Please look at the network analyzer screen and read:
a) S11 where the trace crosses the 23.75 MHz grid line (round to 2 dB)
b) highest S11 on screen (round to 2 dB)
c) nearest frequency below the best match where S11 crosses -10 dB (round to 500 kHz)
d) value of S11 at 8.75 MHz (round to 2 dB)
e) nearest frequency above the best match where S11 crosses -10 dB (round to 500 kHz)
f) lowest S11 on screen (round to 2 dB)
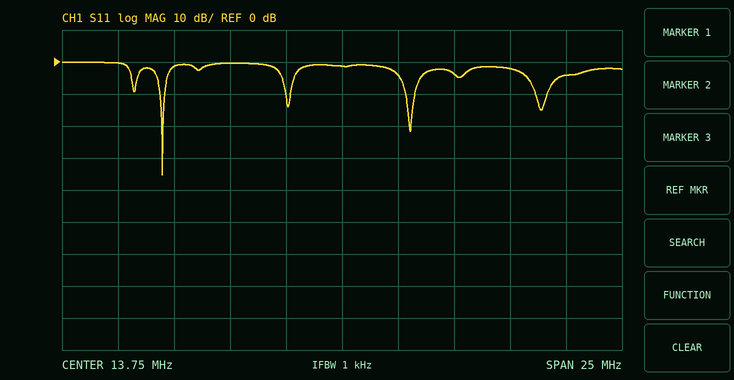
-4 dB
0 dB
5.5 MHz
0 dB
6.0 MHz
-36 dB
